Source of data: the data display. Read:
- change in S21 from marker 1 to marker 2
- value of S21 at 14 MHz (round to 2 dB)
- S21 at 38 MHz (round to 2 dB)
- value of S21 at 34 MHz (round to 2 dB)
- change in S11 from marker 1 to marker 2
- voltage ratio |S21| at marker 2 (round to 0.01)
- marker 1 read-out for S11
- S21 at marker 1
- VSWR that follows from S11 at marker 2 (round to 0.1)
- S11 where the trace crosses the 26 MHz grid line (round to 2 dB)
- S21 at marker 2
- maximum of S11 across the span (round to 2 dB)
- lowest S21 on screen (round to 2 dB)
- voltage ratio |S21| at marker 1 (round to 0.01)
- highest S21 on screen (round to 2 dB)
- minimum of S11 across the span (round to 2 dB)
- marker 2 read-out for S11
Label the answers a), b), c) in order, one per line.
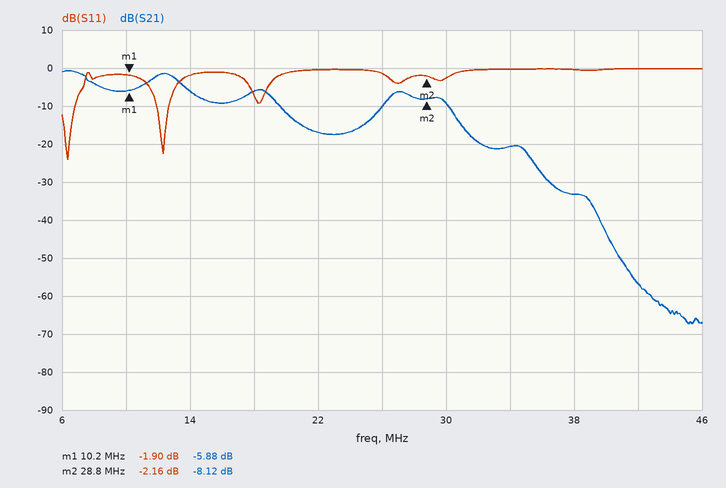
a) -2.24 dB
b) -6 dB
c) -34 dB
d) -20 dB
e) -0.26 dB
f) 0.39
g) -1.90 dB
h) -5.88 dB
i) 8.1
j) -2 dB
k) -8.12 dB
l) 0 dB
m) -68 dB
n) 0.51
o) 0 dB
p) -24 dB
q) -2.16 dB
